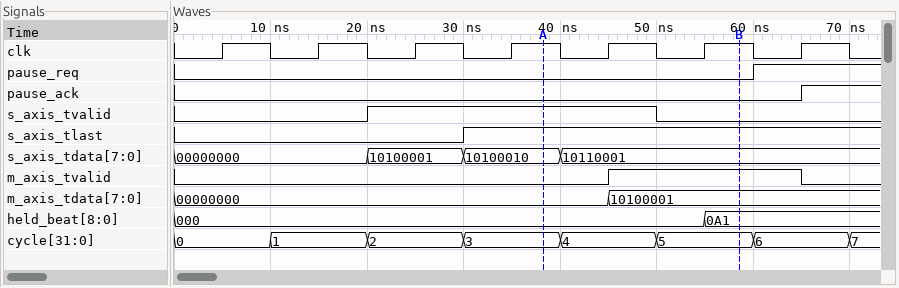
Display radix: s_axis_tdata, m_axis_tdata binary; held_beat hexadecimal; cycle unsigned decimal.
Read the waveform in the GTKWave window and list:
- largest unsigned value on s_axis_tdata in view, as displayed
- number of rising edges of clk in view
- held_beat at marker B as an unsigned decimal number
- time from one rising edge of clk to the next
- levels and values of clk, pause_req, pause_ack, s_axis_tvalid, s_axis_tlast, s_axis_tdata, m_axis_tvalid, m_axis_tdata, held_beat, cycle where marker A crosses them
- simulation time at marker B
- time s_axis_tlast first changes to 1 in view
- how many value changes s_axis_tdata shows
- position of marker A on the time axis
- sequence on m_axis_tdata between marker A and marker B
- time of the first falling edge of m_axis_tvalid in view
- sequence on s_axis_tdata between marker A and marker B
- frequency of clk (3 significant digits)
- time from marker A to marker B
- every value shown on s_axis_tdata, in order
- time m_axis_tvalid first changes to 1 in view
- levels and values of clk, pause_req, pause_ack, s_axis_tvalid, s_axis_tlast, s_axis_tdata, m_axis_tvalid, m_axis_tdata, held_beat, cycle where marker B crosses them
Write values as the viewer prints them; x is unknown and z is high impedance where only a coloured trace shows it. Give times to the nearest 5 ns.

10110001
7
161
10 ns
clk=1, pause_req=0, pause_ack=0, s_axis_tvalid=1, s_axis_tlast=1, s_axis_tdata=10100010, m_axis_tvalid=0, m_axis_tdata=00000000, held_beat=000, cycle=3
60 ns
30 ns
3
40 ns
00000000, 10100001
65 ns
10100010, 10110001
100 MHz
20 ns
00000000, 10100001, 10100010, 10110001
45 ns
clk=1, pause_req=0, pause_ack=0, s_axis_tvalid=0, s_axis_tlast=1, s_axis_tdata=10110001, m_axis_tvalid=1, m_axis_tdata=10100001, held_beat=0A1, cycle=5
